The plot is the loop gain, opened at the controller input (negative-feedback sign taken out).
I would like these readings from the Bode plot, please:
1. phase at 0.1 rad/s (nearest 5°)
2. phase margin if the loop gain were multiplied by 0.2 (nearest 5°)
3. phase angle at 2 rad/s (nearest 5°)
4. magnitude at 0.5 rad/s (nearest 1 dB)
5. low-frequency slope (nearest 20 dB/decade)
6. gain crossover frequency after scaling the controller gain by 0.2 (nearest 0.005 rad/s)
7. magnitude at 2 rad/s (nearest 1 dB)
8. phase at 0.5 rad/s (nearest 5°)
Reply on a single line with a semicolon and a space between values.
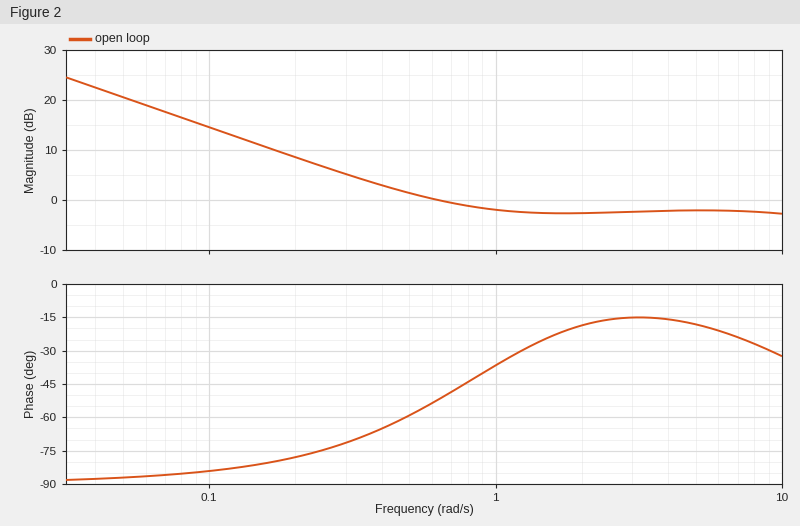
-85°; 95°; -20°; 1 dB; -20 dB/decade; 0.105 rad/s; -3 dB; -60°
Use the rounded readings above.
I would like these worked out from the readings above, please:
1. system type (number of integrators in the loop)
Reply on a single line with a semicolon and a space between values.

1
